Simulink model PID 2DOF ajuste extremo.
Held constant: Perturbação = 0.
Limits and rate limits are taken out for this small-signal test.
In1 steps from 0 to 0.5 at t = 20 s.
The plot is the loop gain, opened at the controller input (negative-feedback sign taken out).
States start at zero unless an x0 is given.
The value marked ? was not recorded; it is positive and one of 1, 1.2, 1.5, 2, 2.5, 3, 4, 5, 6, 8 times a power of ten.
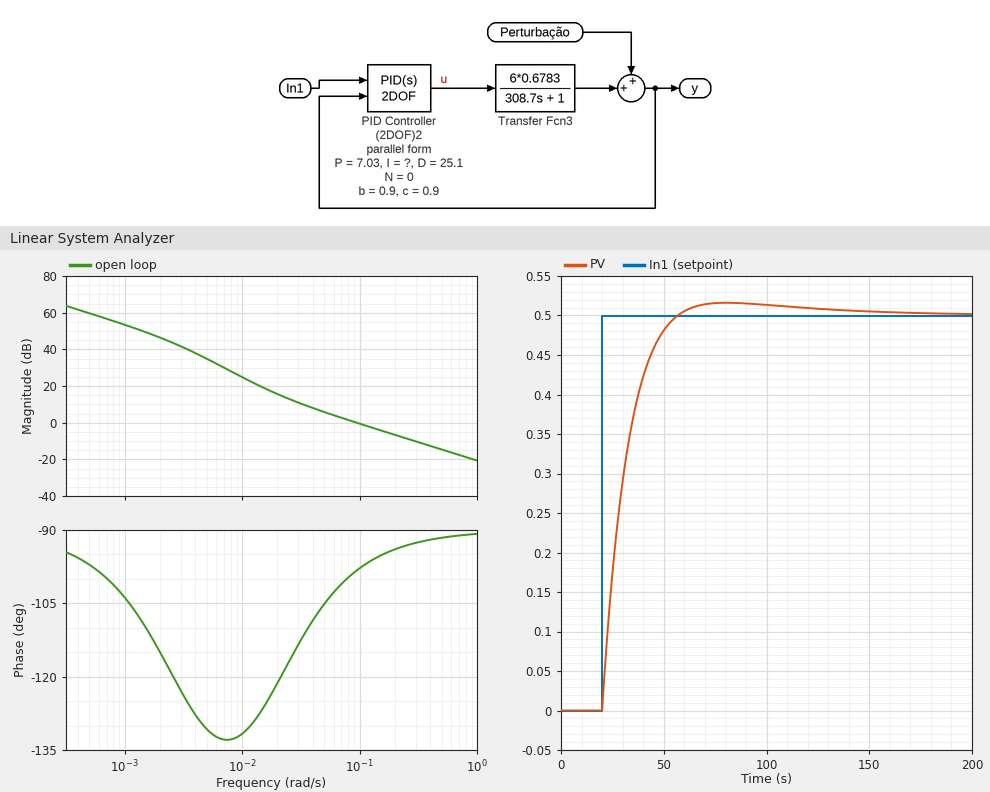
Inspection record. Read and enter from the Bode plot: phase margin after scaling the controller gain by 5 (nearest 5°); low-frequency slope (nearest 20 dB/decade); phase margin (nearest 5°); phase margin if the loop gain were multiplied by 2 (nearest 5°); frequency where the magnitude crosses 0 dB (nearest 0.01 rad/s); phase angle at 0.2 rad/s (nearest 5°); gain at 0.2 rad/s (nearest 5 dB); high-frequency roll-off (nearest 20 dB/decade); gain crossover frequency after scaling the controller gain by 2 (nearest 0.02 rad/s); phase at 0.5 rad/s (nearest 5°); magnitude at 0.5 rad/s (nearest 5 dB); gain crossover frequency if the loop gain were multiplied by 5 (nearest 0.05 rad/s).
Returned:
90°
-20 dB/decade
80°
85°
0.09 rad/s
-95°
-5 dB
-20 dB/decade
0.18 rad/s
-90°
-15 dB
0.45 rad/s
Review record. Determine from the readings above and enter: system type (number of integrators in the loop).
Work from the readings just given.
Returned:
1
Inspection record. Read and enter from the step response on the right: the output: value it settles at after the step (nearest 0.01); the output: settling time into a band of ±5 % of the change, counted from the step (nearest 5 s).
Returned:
0.50
30 s
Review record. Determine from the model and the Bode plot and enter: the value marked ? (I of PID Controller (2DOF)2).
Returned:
0.12
